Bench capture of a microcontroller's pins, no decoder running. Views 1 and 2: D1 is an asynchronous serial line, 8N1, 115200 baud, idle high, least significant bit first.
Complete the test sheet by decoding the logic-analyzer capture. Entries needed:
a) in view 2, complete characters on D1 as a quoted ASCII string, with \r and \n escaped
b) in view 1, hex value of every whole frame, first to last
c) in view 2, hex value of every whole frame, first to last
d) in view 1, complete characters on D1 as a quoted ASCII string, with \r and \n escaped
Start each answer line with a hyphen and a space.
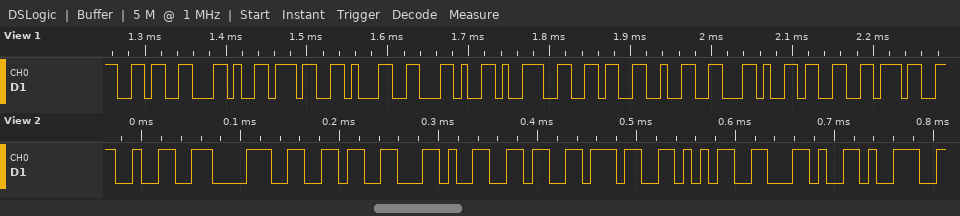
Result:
- "286,675,9"
- 0x36 0x2C 0x37 0x31 0x2C 0x39 0x36 0x32 0x2C 0x33 0x37
- 32 38 36 2C 36 37 35 2C 39
- "6,71,962,37"
